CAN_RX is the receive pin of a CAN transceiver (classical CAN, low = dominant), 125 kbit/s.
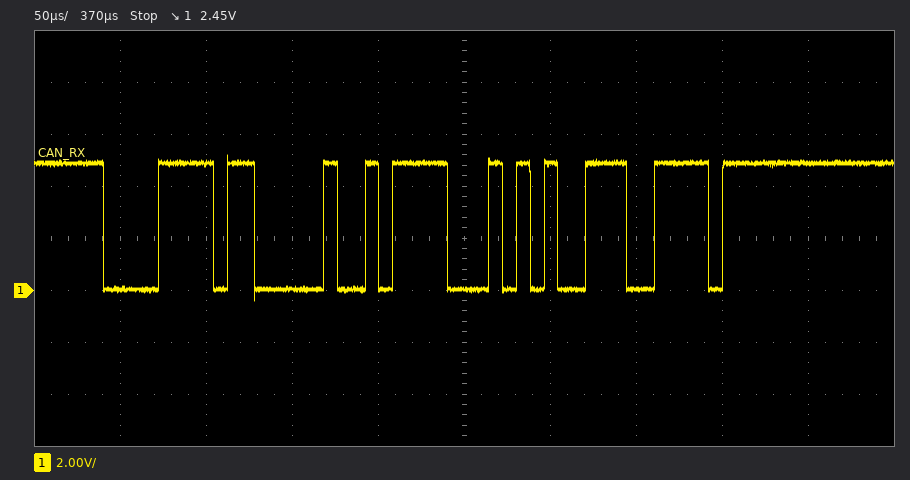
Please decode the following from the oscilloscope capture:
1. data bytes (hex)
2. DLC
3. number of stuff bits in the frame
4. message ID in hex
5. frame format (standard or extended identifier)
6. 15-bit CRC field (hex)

78
1
1
0x0F6
standard
0x54E7
